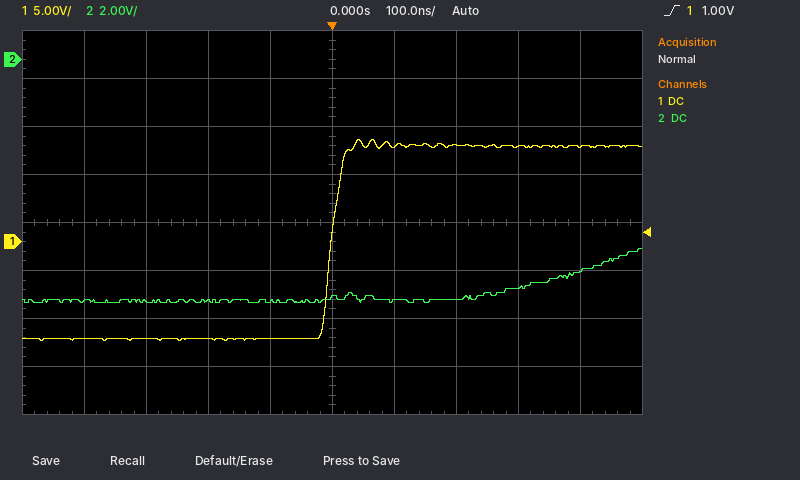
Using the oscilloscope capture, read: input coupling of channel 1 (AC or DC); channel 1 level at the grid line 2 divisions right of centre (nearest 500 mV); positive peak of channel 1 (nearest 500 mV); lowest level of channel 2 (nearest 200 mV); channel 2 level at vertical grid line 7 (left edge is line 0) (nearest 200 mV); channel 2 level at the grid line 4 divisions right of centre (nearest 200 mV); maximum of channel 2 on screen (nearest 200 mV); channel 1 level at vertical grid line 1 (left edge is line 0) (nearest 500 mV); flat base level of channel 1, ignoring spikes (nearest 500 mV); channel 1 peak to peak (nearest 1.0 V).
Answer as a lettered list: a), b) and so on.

a) DC
b) 10.0 V
c) 10.5 V
d) -10.2 V
e) -10.0 V
f) -8.8 V
g) -7.8 V
h) -10.0 V
i) -10.0 V
j) 21.0 V
